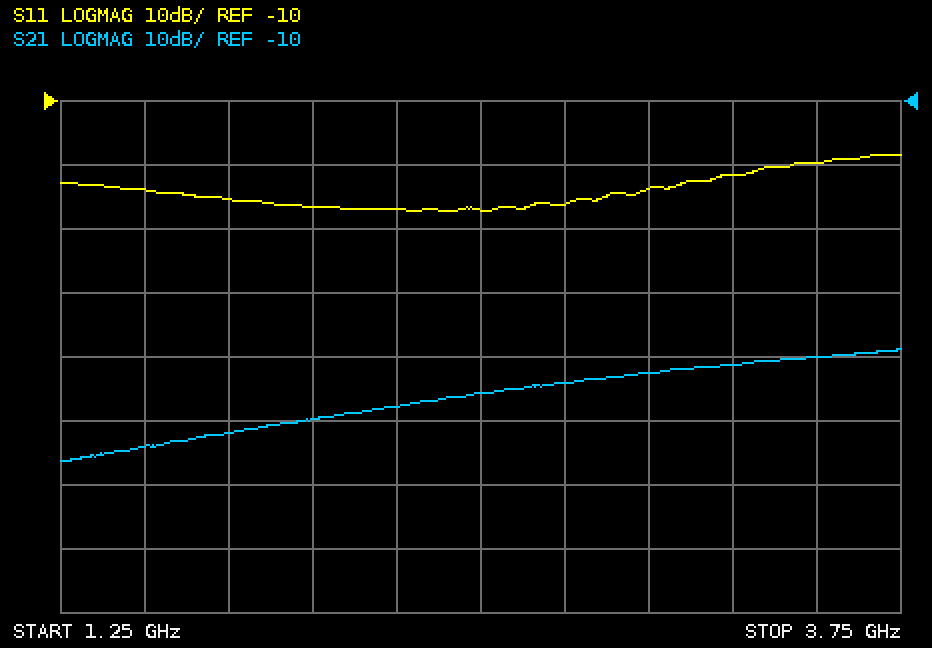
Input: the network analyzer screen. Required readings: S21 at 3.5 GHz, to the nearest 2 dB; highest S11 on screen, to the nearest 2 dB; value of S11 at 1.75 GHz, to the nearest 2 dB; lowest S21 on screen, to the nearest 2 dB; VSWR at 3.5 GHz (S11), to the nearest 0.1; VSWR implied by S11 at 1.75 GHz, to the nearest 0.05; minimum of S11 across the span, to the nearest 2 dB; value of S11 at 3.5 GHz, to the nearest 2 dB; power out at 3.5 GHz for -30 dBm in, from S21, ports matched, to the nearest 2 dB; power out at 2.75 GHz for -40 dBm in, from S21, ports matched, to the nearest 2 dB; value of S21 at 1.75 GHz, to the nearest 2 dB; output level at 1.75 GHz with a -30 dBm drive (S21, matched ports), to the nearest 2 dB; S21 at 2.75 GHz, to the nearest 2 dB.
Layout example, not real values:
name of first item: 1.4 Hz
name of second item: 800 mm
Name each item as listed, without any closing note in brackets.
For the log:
S21 at 3.5 GHz, to the nearest 2 dB: -50 dB
highest S11 on screen, to the nearest 2 dB: -18 dB
value of S11 at 1.75 GHz, to the nearest 2 dB: -26 dB
lowest S21 on screen, to the nearest 2 dB: -66 dB
VSWR at 3.5 GHz (S11), to the nearest 0.1: 1.2
VSWR implied by S11 at 1.75 GHz, to the nearest 0.05: 1.10
minimum of S11 across the span, to the nearest 2 dB: -28 dB
value of S11 at 3.5 GHz, to the nearest 2 dB: -20 dB
power out at 3.5 GHz for -30 dBm in, from S21, ports matched, to the nearest 2 dB: -80 dBm
power out at 2.75 GHz for -40 dBm in, from S21, ports matched, to the nearest 2 dB: -94 dBm
value of S21 at 1.75 GHz, to the nearest 2 dB: -62 dB
output level at 1.75 GHz with a -30 dBm drive (S21, matched ports), to the nearest 2 dB: -92 dBm
S21 at 2.75 GHz, to the nearest 2 dB: -54 dB
